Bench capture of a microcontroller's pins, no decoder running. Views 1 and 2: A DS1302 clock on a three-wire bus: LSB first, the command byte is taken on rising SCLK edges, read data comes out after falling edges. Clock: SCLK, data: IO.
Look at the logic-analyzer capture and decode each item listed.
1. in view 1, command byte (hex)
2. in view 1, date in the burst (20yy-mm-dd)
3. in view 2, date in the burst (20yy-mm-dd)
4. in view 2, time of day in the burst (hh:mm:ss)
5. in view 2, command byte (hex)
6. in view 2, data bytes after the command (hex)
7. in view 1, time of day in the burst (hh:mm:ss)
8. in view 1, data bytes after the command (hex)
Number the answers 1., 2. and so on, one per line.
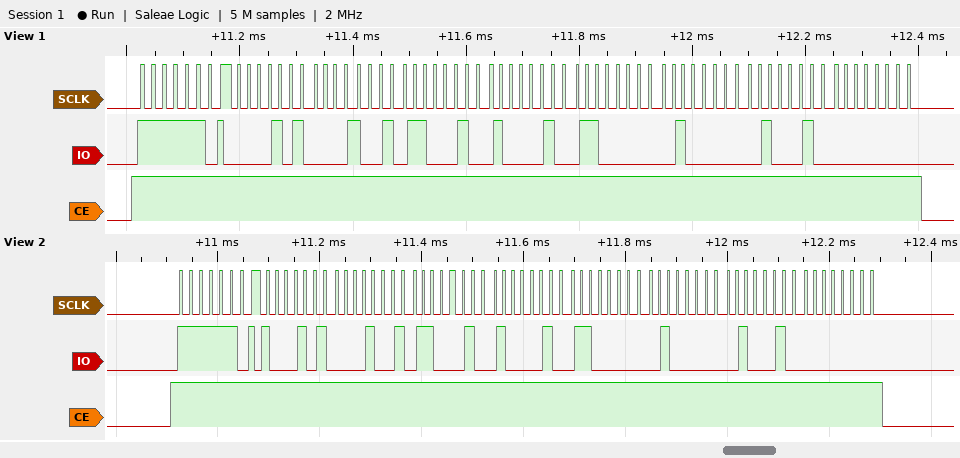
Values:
1. 0xBF
2. 2022-03-21
3. 2022-03-21
4. 23:48:51
5. 0xBF
6. 51 48 23 21 03 02 22 00
7. 23:48:50
8. 50 48 23 21 03 02 22 00
